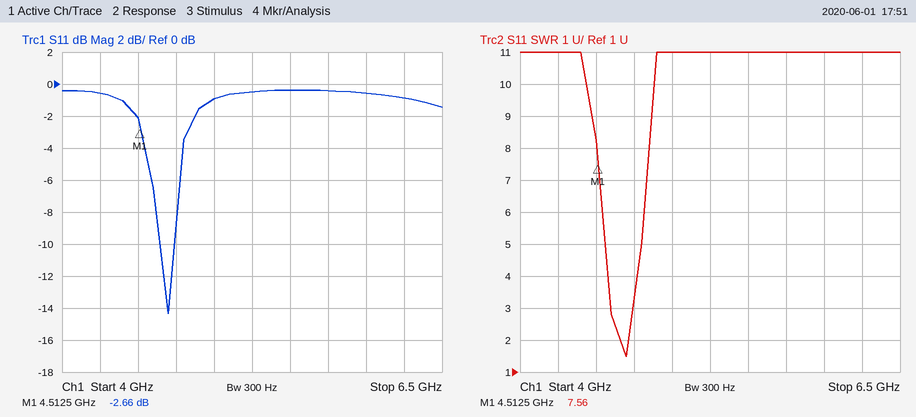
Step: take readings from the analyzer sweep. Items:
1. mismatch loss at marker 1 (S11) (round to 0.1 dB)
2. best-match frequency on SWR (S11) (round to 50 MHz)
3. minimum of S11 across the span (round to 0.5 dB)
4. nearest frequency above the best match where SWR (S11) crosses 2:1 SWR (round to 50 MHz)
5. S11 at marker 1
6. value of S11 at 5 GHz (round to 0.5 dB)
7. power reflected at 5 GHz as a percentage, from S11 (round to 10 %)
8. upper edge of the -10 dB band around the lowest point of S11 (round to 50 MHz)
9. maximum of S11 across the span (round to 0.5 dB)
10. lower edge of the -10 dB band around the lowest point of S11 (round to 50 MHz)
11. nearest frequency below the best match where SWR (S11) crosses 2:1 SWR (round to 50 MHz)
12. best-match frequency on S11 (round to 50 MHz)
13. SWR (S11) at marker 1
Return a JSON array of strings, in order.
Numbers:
["3.4 dB", "4.70 GHz", "-14.5 dB", "4.70 GHz", "-2.66 dB", "-1.0 dB", "80 %", "4.75 GHz", "-0.5 dB", "4.65 GHz", "4.65 GHz", "4.70 GHz", "7.56"]
